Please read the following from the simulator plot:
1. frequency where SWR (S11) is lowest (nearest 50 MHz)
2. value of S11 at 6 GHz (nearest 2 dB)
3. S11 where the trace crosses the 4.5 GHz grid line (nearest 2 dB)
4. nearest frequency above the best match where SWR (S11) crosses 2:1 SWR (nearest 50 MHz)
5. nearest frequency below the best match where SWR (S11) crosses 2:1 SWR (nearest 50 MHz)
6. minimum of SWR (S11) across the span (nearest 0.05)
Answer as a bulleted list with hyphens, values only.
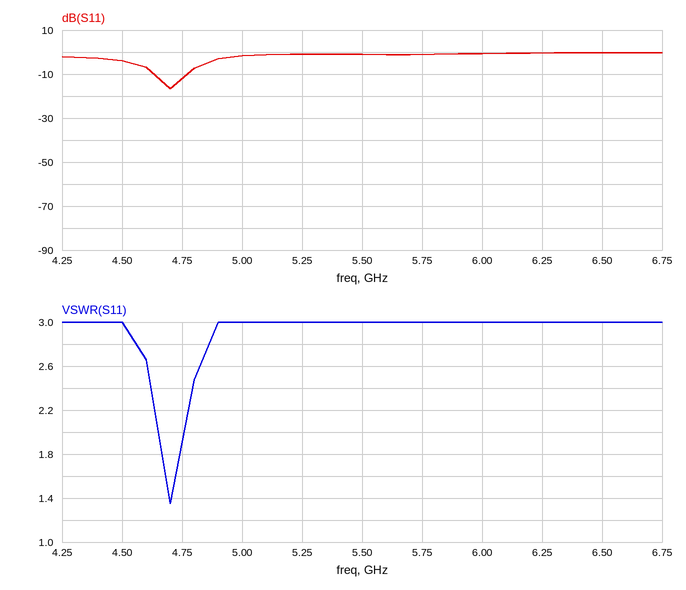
- 4.70 GHz
- 0 dB
- -4 dB
- 4.75 GHz
- 4.65 GHz
- 1.35
